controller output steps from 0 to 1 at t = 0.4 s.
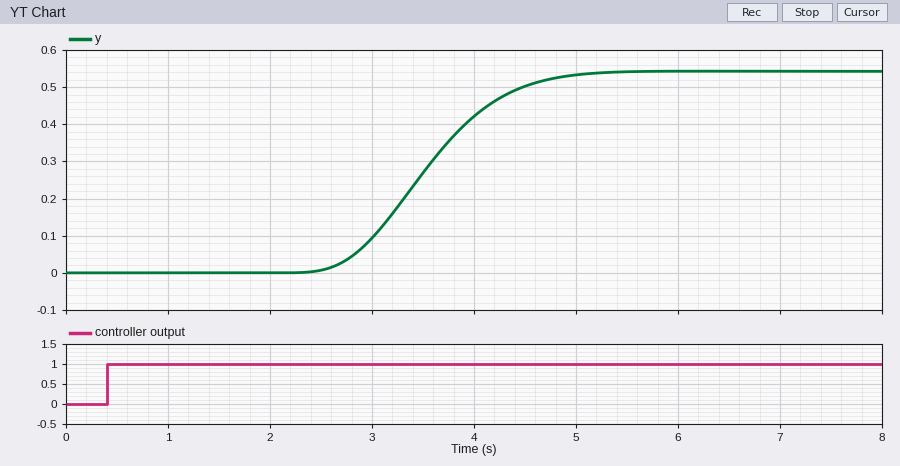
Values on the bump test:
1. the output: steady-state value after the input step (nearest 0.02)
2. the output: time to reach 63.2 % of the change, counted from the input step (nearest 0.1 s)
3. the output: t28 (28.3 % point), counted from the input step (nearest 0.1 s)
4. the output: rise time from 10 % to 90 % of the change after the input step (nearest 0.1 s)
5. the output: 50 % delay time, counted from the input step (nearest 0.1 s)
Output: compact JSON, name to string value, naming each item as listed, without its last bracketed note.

{"the output: steady-state value after the input step": "0.54", "the output: time to reach 63.2 % of the change, counted from the input step": "3.3 s", "the output: t28 (28.3 % point), counted from the input step": "2.8 s", "the output: rise time from 10 % to 90 % of the change after the input step": "1.5 s", "the output: 50 % delay time, counted from the input step": "3.1 s"}
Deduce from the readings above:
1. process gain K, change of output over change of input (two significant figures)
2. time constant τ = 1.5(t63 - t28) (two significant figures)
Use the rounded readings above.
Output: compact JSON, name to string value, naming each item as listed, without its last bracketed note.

{"process gain K, change of output over change of input": "0.54", "time constant τ = 1.5(t63 - t28)": "0.75 s"}
